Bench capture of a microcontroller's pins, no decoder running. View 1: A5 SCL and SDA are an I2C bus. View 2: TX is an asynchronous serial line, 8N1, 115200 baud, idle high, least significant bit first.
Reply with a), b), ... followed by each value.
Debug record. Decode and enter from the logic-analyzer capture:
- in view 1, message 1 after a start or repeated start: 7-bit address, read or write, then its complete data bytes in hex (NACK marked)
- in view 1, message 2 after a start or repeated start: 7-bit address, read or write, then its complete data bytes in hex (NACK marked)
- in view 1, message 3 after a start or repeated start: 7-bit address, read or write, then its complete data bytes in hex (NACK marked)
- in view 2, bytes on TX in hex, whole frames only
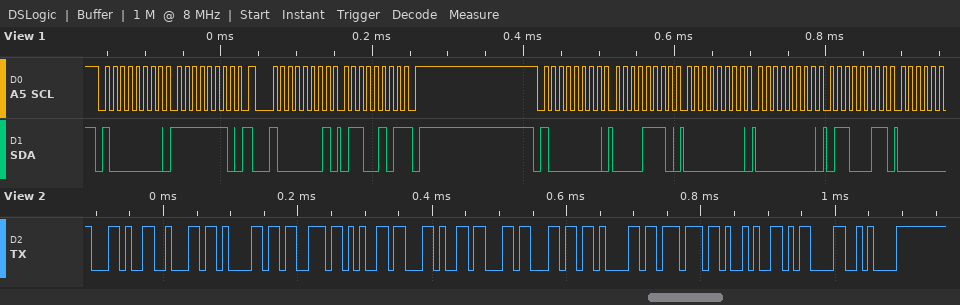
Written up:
a) 0x40 write: FE
b) 0x40 read: 65 NACK
c) 0x40 write: 0E 00 00 63
d) 2C 62 61 73 65 2C 63 6C 61 77 29 0D 0A
